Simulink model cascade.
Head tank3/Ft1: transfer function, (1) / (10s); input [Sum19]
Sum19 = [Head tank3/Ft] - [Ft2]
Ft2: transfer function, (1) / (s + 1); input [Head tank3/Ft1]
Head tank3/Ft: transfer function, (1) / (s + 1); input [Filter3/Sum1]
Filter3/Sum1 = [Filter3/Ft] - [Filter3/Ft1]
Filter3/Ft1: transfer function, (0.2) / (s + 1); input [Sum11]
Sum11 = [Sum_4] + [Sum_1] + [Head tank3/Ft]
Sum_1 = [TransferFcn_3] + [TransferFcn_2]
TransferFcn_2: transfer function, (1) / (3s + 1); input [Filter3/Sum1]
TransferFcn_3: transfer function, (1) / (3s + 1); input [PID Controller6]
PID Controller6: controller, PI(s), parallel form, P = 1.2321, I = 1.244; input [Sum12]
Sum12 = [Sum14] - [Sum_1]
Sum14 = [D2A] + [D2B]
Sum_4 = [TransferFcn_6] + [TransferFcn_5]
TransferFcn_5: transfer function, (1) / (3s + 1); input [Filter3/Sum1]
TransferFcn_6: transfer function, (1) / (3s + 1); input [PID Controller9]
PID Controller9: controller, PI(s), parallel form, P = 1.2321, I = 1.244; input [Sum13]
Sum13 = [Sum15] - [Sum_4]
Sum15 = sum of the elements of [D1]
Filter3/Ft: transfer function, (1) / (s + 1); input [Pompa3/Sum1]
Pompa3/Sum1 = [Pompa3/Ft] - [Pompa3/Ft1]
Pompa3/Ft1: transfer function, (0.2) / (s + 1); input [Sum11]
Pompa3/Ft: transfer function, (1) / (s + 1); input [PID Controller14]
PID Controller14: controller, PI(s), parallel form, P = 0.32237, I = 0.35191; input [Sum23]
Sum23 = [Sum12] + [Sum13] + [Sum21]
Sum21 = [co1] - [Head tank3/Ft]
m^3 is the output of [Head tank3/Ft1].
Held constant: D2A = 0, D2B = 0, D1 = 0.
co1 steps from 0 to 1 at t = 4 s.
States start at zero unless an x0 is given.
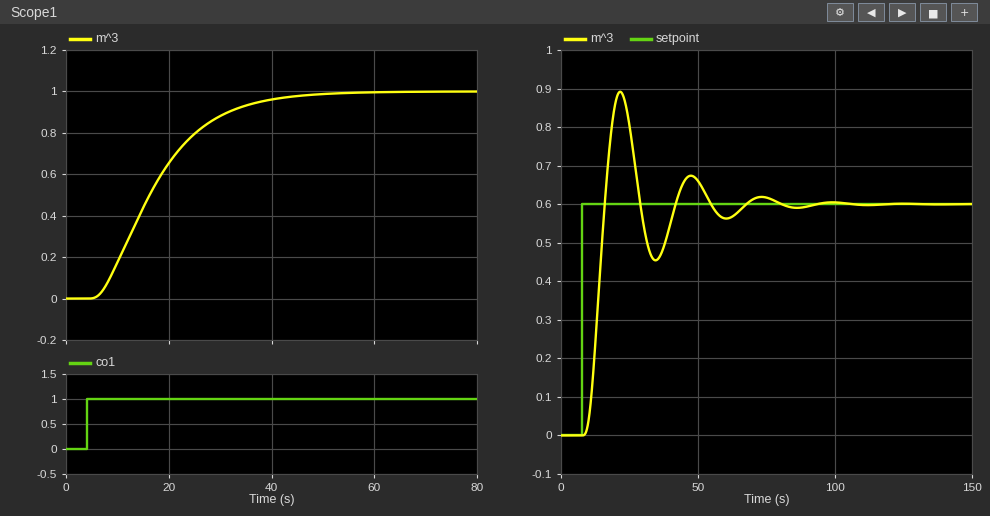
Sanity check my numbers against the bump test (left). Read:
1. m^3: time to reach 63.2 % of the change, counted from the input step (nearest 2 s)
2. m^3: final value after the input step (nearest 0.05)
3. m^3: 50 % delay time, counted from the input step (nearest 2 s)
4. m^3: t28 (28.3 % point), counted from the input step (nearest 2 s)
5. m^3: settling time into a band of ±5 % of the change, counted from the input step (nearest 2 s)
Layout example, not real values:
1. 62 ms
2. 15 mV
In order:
1. 16 s
2. 1.00
3. 12 s
4. 8 s
5. 34 s
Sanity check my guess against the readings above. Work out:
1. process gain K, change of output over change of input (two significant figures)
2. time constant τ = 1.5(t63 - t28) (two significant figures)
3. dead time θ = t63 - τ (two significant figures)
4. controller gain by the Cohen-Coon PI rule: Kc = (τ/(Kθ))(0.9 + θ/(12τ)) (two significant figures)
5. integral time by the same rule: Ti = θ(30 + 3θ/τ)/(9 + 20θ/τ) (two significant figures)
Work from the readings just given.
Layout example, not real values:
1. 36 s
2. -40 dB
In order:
1. 1.0
2. 12 s
3. 4.0 s
4. 2.8
5. 7.9 s
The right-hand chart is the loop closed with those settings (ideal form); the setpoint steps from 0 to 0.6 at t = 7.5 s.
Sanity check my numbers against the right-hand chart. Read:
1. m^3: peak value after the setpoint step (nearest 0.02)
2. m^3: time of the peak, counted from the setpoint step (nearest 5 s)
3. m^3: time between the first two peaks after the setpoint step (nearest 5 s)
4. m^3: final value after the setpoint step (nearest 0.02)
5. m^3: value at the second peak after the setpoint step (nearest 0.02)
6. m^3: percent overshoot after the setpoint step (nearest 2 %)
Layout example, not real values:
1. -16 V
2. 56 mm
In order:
1. 0.90
2. 15 s
3. 25 s
4. 0.60
5. 0.68
6. 48 %
